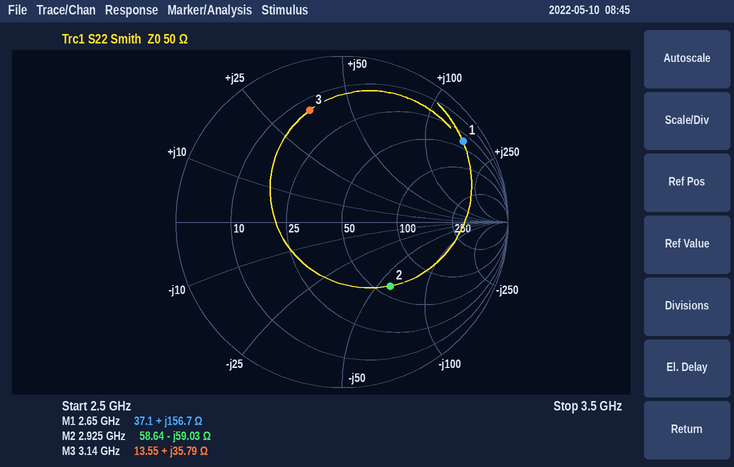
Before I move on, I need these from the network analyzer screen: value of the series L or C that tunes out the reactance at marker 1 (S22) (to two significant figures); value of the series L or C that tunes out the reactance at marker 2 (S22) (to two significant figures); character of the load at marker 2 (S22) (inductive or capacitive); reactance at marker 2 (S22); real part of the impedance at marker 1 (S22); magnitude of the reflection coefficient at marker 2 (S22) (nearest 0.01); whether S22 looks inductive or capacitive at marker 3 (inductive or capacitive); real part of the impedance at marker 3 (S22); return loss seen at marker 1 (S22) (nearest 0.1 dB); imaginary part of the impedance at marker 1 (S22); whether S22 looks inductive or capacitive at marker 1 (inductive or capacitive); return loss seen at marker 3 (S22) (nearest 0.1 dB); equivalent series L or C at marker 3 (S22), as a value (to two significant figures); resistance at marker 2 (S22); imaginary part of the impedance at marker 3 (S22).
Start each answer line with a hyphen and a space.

- 380 fF
- 3.2 nH
- capacitive
- -59.03 Ω
- 37.1 Ω
- 0.48
- inductive
- 13.55 Ω
- 1.1 dB
- +156.7 Ω
- inductive
- 3.1 dB
- 1.8 nH
- 58.64 Ω
- +35.79 Ω
